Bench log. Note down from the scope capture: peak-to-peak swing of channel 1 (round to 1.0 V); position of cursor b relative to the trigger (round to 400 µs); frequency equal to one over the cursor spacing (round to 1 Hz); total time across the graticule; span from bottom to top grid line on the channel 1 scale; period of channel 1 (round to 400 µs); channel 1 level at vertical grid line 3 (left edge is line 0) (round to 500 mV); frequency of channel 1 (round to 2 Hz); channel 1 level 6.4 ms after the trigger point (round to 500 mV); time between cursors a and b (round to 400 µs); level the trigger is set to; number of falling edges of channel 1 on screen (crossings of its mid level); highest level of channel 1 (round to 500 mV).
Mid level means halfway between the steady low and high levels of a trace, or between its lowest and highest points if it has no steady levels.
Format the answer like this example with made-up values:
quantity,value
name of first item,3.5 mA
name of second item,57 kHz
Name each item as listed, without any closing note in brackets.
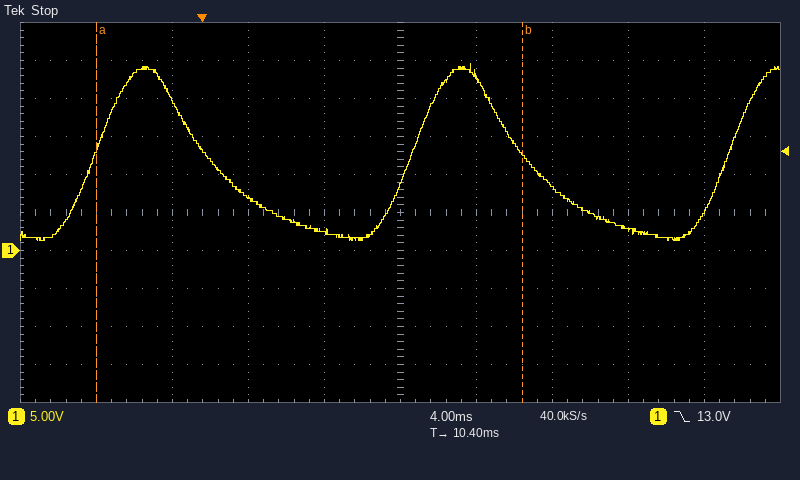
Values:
quantity,value
peak-to-peak swing of channel 1,23.0 V
position of cursor b relative to the trigger,+16.8 ms
frequency equal to one over the cursor spacing,45 Hz
total time across the graticule,40 ms
span from bottom to top grid line on the channel 1 scale,50 V
period of channel 1,16.8 ms
channel 1 level at vertical grid line 3 (left edge is line 0),7.0 V
frequency of channel 1,60 Hz
channel 1 level 6.4 ms after the trigger point,2.5 V
time between cursors a and b,22.4 ms
level the trigger is set to,13.0 V
number of falling edges of channel 1 on screen,2
highest level of channel 1,24.5 V
